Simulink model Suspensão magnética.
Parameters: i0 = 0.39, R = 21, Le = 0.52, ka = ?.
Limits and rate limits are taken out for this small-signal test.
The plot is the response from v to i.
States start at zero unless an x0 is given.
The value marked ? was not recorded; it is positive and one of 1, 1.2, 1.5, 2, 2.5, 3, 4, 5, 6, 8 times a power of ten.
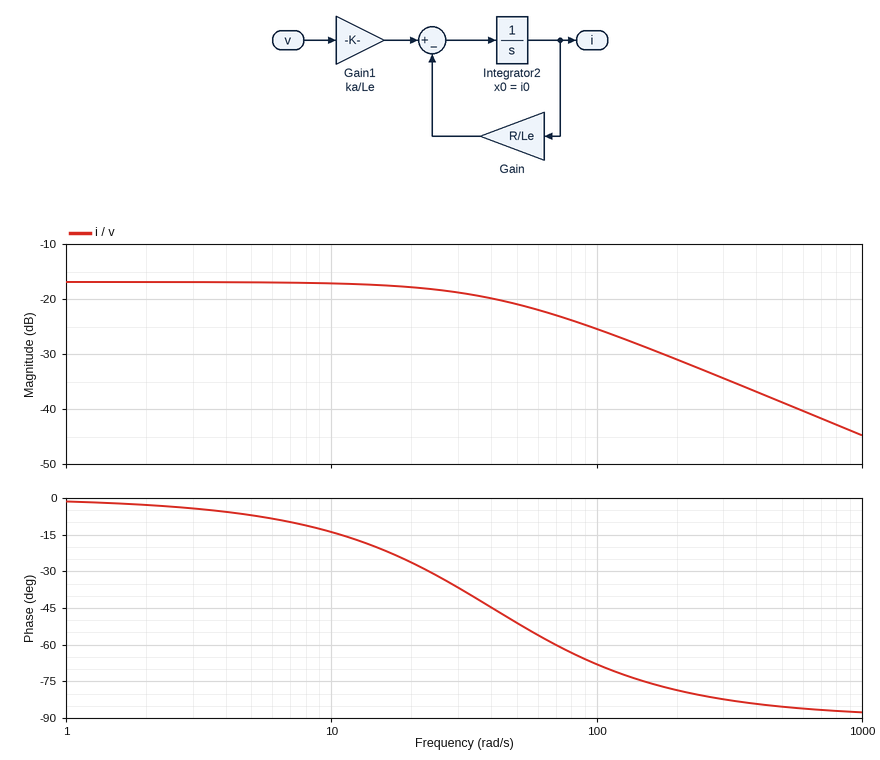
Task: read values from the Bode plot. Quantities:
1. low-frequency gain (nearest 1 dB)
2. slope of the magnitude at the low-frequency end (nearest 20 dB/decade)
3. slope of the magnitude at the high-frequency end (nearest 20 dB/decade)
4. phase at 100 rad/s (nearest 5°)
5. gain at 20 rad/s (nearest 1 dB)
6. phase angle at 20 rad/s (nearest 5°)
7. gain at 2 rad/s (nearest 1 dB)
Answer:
-17 dB
0 dB/decade
-20 dB/decade
-70°
-18 dB
-25°
-17 dB
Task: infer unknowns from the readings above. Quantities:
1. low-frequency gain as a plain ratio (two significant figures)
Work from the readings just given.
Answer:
0.14
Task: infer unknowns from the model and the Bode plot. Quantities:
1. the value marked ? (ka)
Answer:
3
